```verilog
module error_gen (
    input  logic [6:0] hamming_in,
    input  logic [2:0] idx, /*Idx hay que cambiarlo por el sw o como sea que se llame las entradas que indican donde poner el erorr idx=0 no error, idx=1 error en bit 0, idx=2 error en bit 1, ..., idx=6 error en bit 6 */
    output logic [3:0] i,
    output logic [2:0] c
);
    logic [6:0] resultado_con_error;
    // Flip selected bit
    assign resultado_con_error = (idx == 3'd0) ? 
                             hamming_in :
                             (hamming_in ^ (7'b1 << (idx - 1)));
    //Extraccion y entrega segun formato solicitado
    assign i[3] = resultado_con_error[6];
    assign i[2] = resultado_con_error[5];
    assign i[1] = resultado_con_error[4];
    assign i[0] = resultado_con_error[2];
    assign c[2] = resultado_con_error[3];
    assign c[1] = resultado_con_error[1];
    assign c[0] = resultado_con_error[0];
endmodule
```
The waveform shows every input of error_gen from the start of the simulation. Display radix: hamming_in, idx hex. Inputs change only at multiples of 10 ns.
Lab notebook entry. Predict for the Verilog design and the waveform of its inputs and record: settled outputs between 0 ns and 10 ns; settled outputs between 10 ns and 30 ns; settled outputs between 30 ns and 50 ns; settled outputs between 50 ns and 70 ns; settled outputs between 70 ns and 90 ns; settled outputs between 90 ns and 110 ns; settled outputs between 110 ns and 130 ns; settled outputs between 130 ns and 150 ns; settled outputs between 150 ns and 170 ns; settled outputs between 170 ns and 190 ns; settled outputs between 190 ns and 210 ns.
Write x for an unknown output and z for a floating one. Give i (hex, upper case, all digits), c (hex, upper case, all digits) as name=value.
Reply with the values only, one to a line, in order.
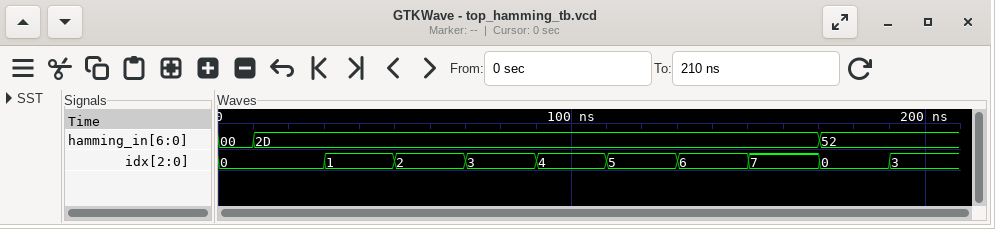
i=0, c=0
i=5, c=5
i=5, c=4
i=5, c=7
i=4, c=5
i=5, c=1
i=7, c=5
i=1, c=5
i=D, c=5
i=A, c=2
i=B, c=2
